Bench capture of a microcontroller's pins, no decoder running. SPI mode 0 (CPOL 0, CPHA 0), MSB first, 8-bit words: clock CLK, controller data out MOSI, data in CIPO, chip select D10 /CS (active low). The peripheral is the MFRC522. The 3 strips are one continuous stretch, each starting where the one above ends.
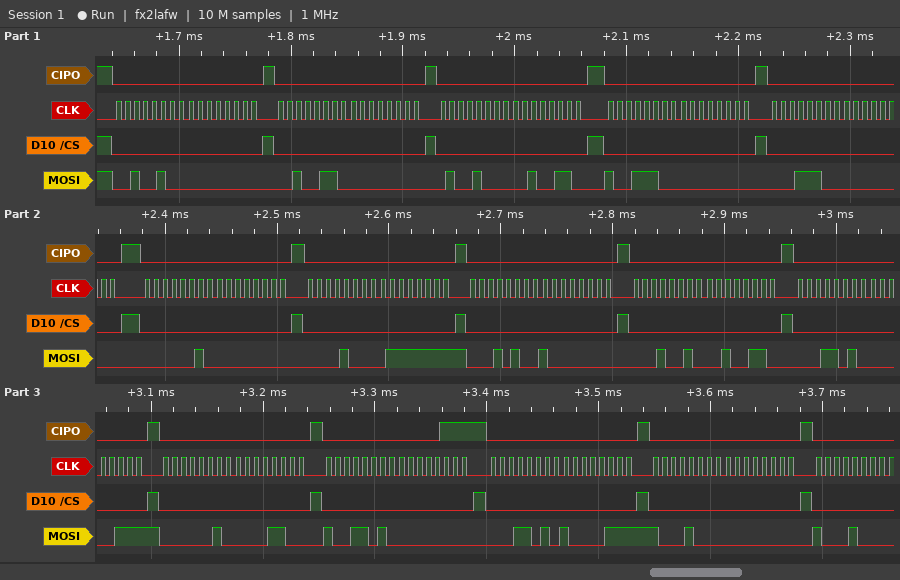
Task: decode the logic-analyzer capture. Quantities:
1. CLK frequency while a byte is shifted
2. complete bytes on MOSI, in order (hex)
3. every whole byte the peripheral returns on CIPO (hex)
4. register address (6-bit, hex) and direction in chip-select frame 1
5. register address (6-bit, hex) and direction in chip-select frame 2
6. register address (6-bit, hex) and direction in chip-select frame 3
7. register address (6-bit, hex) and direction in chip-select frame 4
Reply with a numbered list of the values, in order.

1. 125 kHz
2. 24 00 26 00 48 26 9C 00 1C 00 02 00 08 7F 14 80 12 26 1A 07 02 0C 9A 00 1A 87 88 00 88
3. 00 00 00 00 00 00 00 00 00 00 00 00 00 00 00 00 00 00 00 00 00 00 00 07 00 00 00 00 00
4. 0x12 write
5. 0x13 write
6. 0x24 write
7. 0x0E read
